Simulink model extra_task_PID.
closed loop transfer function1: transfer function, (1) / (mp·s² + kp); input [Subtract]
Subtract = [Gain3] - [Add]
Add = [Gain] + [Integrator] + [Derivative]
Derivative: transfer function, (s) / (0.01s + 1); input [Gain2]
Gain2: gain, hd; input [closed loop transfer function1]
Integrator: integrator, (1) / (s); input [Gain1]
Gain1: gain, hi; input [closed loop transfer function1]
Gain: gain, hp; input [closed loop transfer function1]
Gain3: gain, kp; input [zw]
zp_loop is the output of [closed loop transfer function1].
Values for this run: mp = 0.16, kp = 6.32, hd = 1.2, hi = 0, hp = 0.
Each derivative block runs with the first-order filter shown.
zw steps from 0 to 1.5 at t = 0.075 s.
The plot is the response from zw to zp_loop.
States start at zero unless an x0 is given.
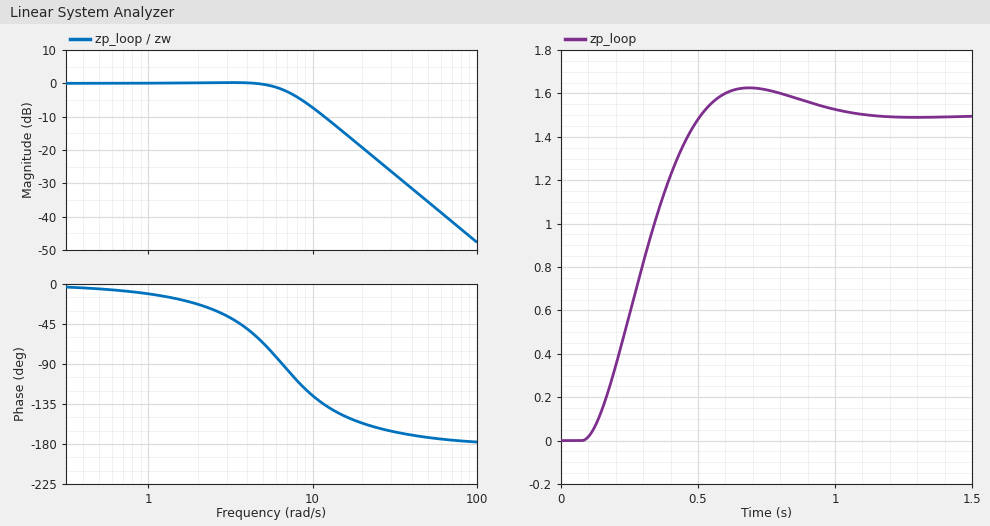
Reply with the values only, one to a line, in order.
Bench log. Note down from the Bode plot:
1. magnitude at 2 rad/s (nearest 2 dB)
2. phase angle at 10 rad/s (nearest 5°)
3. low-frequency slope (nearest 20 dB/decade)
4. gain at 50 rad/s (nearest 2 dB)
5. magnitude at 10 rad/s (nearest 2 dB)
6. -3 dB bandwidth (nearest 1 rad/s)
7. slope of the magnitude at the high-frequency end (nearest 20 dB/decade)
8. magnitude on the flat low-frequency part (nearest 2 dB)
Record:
0 dB
-125°
0 dB/decade
-36 dB
-8 dB
7 rad/s
-40 dB/decade
0 dB
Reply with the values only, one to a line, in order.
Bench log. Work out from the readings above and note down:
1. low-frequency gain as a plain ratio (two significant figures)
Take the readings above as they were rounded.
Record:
1.0
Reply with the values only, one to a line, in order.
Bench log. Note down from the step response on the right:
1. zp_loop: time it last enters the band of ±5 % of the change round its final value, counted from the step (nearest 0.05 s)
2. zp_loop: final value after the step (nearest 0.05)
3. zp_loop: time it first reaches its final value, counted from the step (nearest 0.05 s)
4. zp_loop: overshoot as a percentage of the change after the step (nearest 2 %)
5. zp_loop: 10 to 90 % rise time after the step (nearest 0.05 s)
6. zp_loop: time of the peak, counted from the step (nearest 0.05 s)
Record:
0.80 s
1.50
0.45 s
8 %
0.30 s
0.60 s
